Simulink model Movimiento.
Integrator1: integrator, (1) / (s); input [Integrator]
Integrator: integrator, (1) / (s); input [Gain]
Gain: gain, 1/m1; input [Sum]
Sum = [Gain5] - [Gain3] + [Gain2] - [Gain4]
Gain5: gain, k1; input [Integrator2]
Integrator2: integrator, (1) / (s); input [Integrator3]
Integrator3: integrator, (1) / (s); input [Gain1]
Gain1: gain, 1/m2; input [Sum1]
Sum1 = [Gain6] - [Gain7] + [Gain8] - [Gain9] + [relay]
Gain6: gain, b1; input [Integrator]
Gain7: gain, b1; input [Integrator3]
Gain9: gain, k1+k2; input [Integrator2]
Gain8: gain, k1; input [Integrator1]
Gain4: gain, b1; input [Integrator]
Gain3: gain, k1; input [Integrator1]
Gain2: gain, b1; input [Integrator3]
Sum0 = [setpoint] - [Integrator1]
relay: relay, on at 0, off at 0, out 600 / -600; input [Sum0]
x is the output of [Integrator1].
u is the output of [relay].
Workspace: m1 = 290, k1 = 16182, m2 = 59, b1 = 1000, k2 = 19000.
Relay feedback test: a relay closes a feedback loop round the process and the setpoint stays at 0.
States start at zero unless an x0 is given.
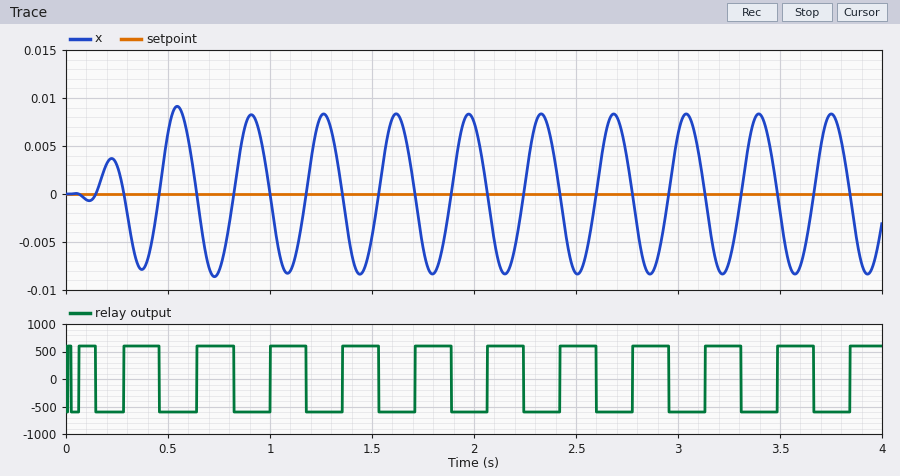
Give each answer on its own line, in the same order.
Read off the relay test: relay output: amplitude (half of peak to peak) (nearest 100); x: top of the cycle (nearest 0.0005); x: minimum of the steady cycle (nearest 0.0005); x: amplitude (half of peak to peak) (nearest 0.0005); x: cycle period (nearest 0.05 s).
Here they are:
600
0.0085
-0.0085
0.0085
0.35 s
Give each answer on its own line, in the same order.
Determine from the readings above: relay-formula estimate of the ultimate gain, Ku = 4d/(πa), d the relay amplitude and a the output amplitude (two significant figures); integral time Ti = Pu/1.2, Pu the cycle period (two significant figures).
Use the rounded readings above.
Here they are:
90000
0.29 s
